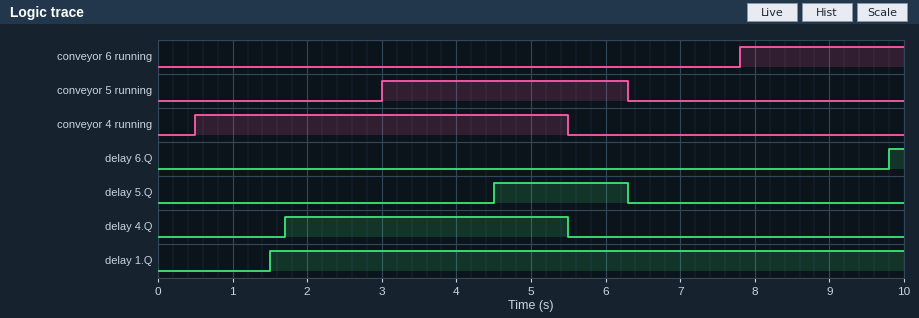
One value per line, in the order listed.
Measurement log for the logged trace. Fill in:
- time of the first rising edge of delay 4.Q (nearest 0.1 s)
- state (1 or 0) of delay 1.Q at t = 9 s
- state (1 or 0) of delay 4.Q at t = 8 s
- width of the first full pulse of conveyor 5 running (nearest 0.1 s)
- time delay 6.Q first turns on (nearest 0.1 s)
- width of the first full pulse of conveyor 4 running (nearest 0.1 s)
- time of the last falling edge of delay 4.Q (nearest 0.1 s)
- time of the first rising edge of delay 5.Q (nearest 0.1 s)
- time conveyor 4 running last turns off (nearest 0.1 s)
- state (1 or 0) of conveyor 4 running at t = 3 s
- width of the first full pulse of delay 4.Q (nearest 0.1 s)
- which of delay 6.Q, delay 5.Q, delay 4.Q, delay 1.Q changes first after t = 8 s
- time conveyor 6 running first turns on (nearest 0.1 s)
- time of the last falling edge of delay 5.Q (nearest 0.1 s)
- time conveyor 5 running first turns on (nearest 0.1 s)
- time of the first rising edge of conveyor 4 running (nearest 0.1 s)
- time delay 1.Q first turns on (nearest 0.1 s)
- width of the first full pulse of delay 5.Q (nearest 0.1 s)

1.7 s
1
0
3.3 s
9.8 s
5.0 s
5.5 s
4.5 s
5.5 s
1
3.8 s
delay 6.Q
7.8 s
6.3 s
3.0 s
0.5 s
1.5 s
1.8 s
